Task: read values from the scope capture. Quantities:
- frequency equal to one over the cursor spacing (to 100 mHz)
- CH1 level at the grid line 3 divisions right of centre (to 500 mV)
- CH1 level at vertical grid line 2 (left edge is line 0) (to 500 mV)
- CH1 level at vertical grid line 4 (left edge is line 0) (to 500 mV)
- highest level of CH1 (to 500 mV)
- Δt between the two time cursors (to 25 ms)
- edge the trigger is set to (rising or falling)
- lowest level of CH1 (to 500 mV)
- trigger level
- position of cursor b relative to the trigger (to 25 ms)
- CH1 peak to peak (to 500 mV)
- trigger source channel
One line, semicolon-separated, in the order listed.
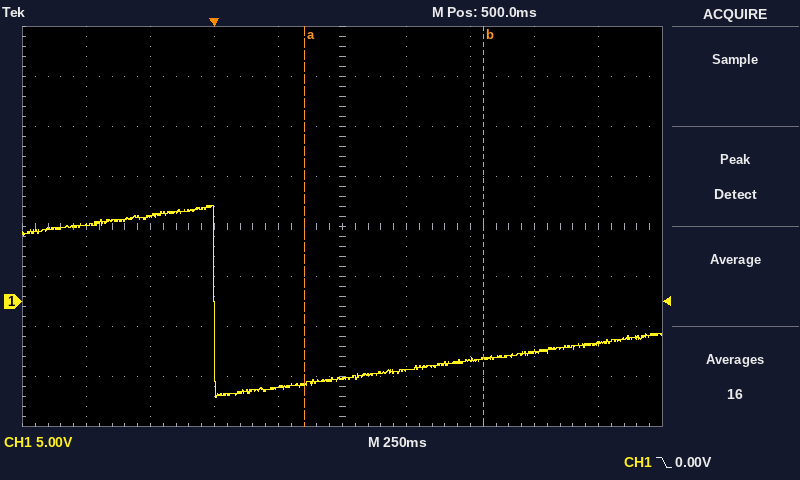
1.4 Hz; -5.0 V; 8.5 V; -8.5 V; 9.5 V; 700 ms; falling; -9.5 V; 0.00 V; +1.050 s; 19.0 V; CH1
